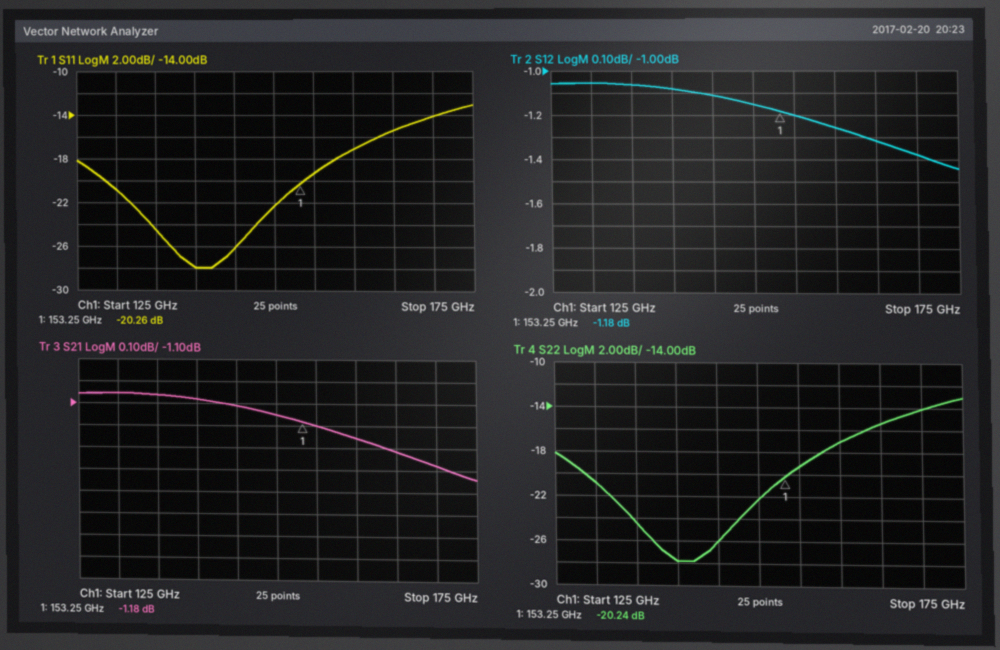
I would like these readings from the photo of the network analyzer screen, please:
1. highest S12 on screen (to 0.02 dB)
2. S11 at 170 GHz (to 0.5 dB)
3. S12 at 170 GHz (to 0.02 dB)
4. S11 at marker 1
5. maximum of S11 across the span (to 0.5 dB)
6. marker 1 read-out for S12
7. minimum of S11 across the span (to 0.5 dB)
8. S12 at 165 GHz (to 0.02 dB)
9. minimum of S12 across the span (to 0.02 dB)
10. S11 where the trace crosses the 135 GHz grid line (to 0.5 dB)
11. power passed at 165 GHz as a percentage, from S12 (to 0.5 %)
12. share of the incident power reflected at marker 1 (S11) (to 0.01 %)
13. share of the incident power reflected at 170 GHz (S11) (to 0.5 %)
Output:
-1.06 dB
-14.0 dB
-1.38 dB
-20.26 dB
-13.0 dB
-1.18 dB
-28.0 dB
-1.32 dB
-1.44 dB
-24.5 dB
74.0 %
0.94 %
4.0 %
